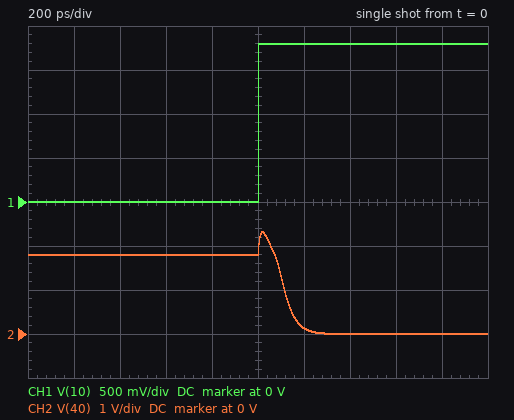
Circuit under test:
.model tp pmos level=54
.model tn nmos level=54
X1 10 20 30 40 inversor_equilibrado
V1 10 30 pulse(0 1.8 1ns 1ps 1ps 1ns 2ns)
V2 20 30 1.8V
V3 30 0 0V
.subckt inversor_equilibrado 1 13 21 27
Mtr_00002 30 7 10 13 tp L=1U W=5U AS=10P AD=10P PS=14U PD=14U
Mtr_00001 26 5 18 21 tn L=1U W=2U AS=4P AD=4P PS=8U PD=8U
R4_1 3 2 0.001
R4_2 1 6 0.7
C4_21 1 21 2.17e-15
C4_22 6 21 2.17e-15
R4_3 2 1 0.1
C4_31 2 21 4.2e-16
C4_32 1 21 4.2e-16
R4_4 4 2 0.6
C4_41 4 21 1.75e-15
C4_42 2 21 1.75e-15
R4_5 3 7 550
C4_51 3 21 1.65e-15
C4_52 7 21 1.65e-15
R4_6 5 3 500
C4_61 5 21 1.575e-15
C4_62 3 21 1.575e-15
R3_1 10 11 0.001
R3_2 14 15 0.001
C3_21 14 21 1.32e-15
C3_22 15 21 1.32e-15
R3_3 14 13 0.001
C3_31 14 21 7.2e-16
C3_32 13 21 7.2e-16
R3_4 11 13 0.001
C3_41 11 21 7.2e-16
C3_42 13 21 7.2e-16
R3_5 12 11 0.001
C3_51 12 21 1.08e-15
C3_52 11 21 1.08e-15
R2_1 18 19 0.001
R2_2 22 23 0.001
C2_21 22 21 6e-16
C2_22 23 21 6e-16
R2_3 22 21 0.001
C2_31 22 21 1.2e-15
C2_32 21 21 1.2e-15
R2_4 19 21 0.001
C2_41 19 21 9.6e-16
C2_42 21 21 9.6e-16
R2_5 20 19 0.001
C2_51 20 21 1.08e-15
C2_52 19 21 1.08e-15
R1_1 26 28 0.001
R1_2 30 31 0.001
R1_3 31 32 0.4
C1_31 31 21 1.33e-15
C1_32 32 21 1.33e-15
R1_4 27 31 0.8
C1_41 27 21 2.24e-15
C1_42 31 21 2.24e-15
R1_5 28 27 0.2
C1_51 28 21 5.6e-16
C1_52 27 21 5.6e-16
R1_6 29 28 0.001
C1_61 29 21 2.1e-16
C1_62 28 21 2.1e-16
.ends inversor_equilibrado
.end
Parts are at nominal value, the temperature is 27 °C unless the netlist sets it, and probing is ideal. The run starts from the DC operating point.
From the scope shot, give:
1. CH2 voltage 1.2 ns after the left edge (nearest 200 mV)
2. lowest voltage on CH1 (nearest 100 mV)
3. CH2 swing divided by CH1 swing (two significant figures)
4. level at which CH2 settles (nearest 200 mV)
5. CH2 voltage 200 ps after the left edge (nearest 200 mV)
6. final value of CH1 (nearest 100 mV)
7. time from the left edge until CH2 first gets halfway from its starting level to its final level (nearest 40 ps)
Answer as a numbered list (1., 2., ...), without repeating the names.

1. 200 mV
2. 0 V
3. 1.3
4. 0 V
5. 1.8 V
6. 1.8 V
7. 1.12 ns
